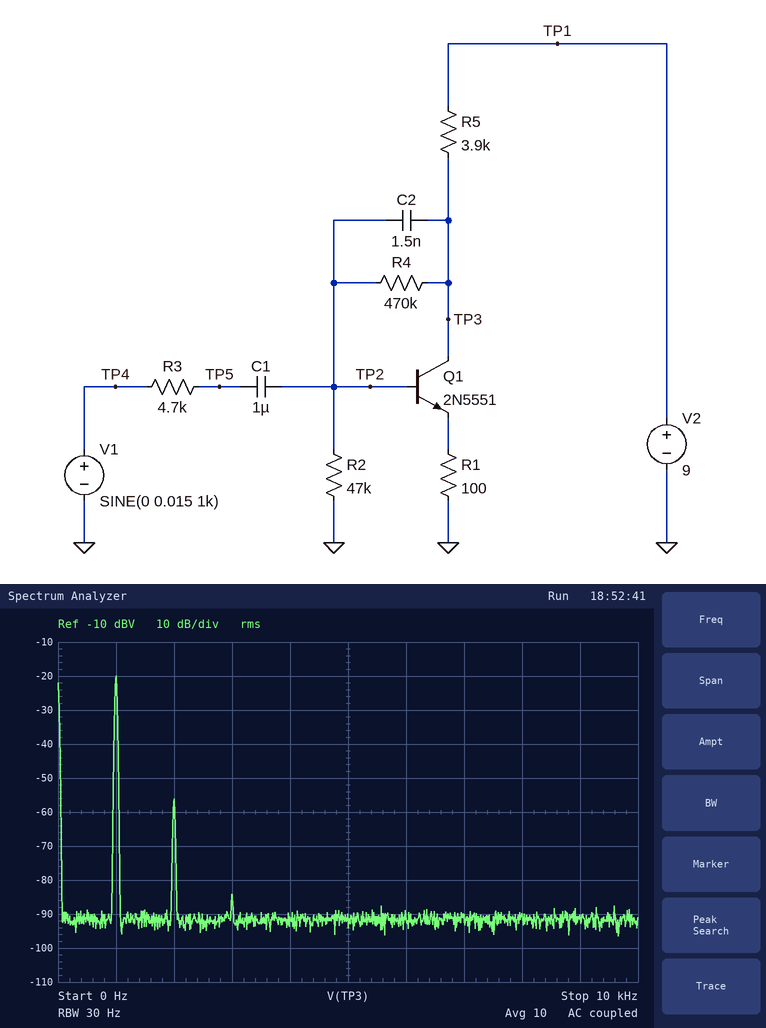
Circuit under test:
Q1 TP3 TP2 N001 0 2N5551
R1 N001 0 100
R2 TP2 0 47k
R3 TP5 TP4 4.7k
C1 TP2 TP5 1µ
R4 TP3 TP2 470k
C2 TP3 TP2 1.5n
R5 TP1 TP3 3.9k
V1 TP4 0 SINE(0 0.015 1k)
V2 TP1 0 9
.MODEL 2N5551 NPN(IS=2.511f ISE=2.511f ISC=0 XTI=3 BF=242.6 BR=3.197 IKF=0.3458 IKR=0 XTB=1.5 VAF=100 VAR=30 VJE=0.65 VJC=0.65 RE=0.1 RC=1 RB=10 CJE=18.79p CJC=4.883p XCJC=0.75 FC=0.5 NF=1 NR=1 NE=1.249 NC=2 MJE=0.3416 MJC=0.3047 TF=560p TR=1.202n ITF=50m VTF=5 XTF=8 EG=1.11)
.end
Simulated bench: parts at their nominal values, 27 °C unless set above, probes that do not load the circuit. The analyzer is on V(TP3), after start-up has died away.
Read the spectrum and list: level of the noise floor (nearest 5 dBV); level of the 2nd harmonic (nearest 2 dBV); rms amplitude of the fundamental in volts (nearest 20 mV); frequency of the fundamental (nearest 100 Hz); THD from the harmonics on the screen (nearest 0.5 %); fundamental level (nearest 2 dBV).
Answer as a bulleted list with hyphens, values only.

- -90 dBV
- -56 dBV
- 100 mV
- 1.0 kHz
- 1.5 %
- -20 dBV
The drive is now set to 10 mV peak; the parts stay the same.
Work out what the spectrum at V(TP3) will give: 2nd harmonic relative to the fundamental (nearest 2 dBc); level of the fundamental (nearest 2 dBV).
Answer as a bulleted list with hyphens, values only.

- -40 dBc
- -24 dBV
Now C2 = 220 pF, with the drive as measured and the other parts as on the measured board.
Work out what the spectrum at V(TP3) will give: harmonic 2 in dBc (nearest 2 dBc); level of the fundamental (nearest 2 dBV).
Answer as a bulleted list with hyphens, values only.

- -32 dBc
- -18 dBV
